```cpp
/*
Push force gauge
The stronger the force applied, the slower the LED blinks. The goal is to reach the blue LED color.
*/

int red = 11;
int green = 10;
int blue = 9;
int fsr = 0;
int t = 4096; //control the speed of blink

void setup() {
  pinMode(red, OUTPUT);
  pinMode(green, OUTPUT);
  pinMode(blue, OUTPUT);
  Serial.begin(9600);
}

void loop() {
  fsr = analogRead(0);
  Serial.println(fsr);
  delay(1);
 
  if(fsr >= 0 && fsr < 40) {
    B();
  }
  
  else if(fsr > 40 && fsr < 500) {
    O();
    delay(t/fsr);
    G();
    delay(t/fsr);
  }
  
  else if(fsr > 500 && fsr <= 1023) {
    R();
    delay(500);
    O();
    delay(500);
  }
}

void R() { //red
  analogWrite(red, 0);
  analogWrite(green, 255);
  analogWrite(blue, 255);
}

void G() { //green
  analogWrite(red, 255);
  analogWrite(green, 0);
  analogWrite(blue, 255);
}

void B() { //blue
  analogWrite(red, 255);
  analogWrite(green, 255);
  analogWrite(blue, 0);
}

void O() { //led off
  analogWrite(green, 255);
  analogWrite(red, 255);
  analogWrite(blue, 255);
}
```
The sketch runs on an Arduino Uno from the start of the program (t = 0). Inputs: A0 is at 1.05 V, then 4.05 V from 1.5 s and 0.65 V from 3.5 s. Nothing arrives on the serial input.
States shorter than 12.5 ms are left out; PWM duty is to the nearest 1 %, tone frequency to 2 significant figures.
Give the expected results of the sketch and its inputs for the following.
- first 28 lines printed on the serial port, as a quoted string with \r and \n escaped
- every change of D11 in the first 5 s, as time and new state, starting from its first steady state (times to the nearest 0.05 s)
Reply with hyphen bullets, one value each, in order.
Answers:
- "215\r\n215\r\n215\r\n215\r\n215\r\n215\r\n215\r\n215\r\n215\r\n215\r\n215\r\n215\r\n215\r\n215\r\n215\r\n215\r\n215\r\n215\r\n215\r\n215\r\n215\r\n215\r\n215\r\n215\r\n215\r\n215\r\n215\r\n215\r\n"
- 0 s high; 1.55 s low; 2.05 s high; 2.55 s low; 3.05 s high
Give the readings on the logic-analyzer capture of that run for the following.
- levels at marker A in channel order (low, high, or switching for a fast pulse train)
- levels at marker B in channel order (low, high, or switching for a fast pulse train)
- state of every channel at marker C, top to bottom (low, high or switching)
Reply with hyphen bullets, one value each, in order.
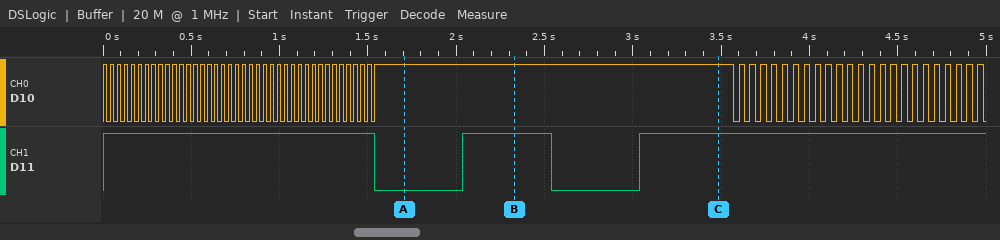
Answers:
- D10 high, D11 low
- D10 high, D11 high
- D10 high, D11 high
